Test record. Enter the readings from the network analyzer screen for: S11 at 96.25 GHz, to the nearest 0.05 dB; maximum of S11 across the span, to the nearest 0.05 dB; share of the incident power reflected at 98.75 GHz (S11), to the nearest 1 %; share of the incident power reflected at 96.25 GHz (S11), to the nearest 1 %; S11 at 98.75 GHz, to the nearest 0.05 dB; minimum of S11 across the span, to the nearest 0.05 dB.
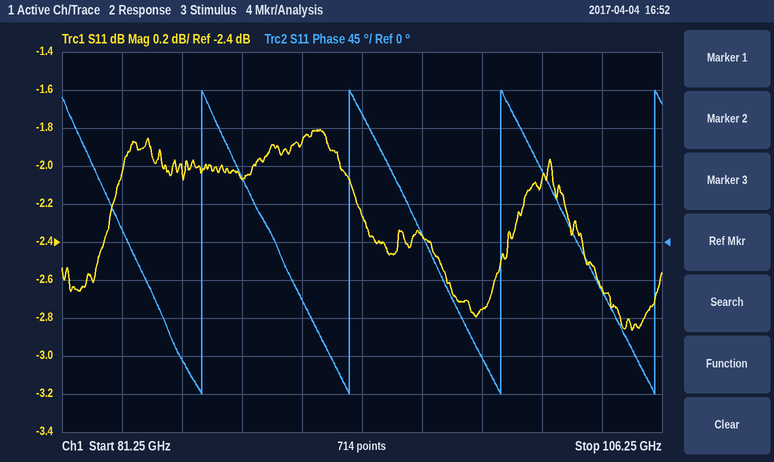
-2.35 dB
-1.80 dB
53 %
58 %
-2.75 dB
-2.85 dB
